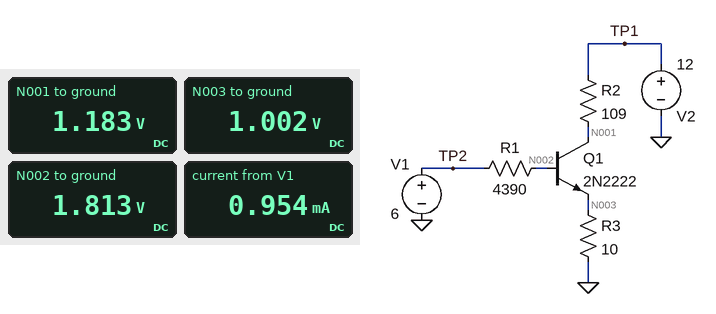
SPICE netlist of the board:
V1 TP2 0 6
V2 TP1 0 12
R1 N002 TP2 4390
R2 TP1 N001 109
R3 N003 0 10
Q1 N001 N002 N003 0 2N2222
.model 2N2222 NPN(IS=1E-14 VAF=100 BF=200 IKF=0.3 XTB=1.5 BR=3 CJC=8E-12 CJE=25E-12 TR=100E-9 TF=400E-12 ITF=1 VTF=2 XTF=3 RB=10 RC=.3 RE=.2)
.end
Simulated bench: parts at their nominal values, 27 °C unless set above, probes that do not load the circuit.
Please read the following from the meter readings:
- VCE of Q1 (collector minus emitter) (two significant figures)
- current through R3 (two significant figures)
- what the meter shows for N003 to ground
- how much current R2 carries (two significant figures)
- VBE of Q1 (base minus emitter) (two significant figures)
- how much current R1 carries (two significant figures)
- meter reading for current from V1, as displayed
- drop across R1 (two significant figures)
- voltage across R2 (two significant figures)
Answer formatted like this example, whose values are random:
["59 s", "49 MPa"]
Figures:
["180 mV", "100 mA", "1.002 V", "99 mA", "810 mV", "950 µA", "0.954 mA", "4.2 V", "11 V"]
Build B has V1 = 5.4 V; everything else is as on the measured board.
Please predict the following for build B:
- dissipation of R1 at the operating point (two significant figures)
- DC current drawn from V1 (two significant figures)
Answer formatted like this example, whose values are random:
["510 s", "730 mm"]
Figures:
["2.9 mW", "820 µA"]
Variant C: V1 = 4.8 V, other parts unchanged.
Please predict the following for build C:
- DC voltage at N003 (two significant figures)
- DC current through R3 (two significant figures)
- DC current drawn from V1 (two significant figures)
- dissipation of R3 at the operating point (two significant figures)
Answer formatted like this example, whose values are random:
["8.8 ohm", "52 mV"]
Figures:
["990 mV", "99 mA", "680 µA", "99 mW"]
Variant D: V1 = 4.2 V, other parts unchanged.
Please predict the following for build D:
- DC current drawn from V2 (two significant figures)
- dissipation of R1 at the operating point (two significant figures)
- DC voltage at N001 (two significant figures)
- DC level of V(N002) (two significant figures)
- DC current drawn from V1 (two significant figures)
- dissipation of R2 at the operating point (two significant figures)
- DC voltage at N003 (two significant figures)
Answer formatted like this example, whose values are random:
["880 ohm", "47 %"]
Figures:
["89 mA", "1.4 mW", "2.3 V", "1.7 V", "570 µA", "860 mW", "890 mV"]
